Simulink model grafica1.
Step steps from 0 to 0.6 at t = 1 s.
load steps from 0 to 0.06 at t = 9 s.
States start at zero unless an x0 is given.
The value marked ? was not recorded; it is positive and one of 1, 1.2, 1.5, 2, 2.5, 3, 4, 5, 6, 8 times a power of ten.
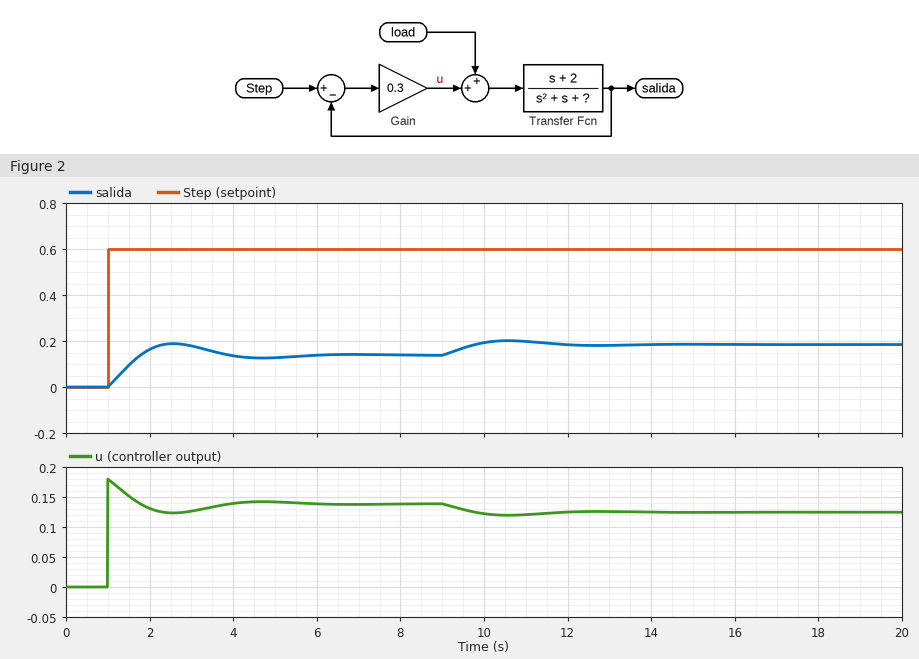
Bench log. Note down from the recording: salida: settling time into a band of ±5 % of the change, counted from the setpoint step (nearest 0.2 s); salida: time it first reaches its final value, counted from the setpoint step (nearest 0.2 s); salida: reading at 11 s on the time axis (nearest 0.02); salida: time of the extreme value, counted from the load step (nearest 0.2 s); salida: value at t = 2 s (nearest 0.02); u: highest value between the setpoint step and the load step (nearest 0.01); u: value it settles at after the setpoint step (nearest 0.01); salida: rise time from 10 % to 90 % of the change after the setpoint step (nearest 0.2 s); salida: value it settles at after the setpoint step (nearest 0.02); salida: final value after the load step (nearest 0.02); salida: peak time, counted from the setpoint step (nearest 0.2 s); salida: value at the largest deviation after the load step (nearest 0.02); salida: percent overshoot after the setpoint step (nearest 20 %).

4.4 s
0.8 s
0.20
1.6 s
0.16
0.18
0.14
0.6 s
0.14
0.18
1.6 s
0.20
40 %
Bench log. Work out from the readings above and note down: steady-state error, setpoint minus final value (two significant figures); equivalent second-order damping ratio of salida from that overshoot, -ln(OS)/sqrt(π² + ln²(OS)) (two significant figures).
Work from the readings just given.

0.46
0.28
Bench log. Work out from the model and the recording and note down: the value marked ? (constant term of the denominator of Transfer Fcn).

2
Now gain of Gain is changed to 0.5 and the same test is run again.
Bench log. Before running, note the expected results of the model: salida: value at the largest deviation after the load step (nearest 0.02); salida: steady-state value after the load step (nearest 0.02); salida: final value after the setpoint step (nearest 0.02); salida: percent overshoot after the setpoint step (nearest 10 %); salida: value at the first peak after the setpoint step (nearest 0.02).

0.26
0.24
0.20
30 %
0.26
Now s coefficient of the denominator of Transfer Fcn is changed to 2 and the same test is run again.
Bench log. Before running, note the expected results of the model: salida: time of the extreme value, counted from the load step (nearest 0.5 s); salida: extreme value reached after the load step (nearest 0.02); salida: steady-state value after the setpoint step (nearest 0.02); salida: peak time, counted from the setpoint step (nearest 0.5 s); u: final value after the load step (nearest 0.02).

2.0 s
0.18
0.14
2.0 s
0.12
